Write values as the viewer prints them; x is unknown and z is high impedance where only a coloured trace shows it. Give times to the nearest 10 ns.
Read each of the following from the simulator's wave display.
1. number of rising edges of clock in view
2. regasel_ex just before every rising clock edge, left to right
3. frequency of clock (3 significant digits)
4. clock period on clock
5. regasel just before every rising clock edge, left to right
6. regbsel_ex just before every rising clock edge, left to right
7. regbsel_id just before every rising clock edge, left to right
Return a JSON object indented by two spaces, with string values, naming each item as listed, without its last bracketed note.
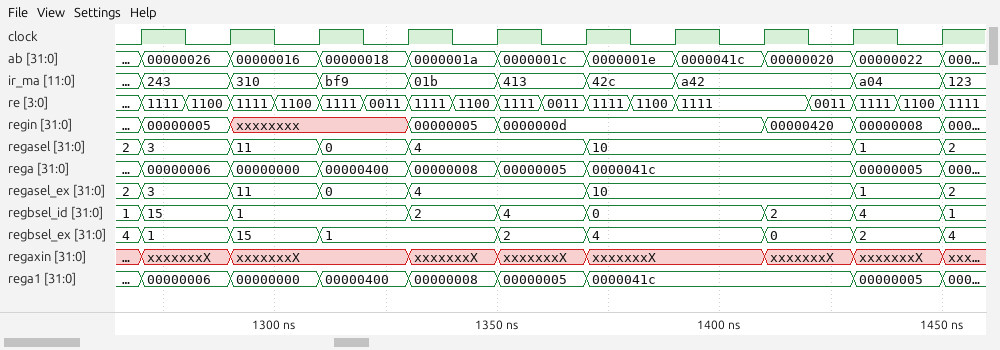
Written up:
{
  "number of rising edges of clock in view": "10",
  "regasel_ex just before every rising clock edge, left to right": "2, 3, 11, 0, 4, 4, 10, 10, 10, 1",
  "frequency of clock": "50.0 MHz",
  "clock period on clock": "20 ns",
  "regasel just before every rising clock edge, left to right": "2, 3, 11, 0, 4, 4, 10, 10, 10, 1",
  "regbsel_ex just before every rising clock edge, left to right": "4, 1, 15, 1, 1, 2, 4, 4, 0, 2",
  "regbsel_id just before every rising clock edge, left to right": "1, 15, 1, 1, 2, 4, 0, 0, 2, 4"
}
